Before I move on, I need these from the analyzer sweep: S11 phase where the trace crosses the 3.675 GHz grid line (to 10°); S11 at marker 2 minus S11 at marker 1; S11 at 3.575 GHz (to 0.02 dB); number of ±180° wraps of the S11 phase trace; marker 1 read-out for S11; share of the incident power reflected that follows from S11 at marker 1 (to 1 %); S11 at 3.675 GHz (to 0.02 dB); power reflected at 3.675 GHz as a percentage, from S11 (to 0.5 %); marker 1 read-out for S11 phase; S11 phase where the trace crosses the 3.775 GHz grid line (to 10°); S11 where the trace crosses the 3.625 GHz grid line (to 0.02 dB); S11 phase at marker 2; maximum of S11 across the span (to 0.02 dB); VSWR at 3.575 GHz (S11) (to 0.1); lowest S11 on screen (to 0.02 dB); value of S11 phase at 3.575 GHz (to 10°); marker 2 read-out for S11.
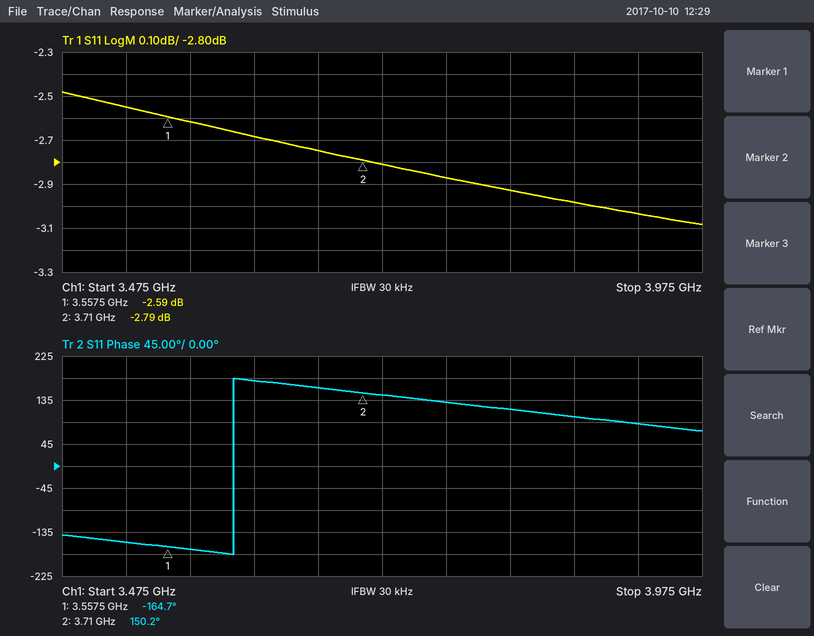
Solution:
160°
-0.20 dB
-2.62 dB
1
-2.59 dB
55 %
-2.74 dB
53.0 %
-164.7°
130°
-2.68 dB
150.2°
-2.48 dB
6.7
-3.08 dB
-170°
-2.79 dB
